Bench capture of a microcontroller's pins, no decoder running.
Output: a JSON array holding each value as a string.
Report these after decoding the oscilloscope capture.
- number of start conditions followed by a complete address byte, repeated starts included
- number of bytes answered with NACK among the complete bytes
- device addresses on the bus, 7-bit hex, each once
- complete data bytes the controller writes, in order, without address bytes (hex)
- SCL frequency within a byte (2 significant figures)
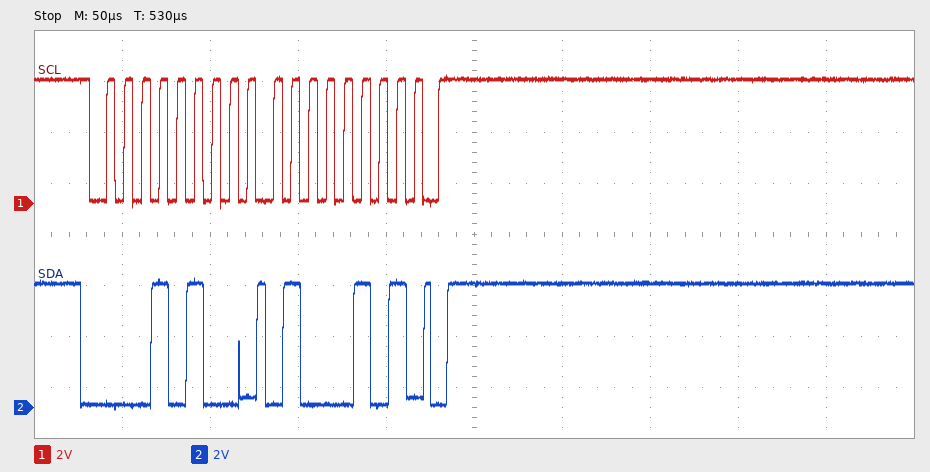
["1", "0", "0x0A", "45", "100 kHz"]
